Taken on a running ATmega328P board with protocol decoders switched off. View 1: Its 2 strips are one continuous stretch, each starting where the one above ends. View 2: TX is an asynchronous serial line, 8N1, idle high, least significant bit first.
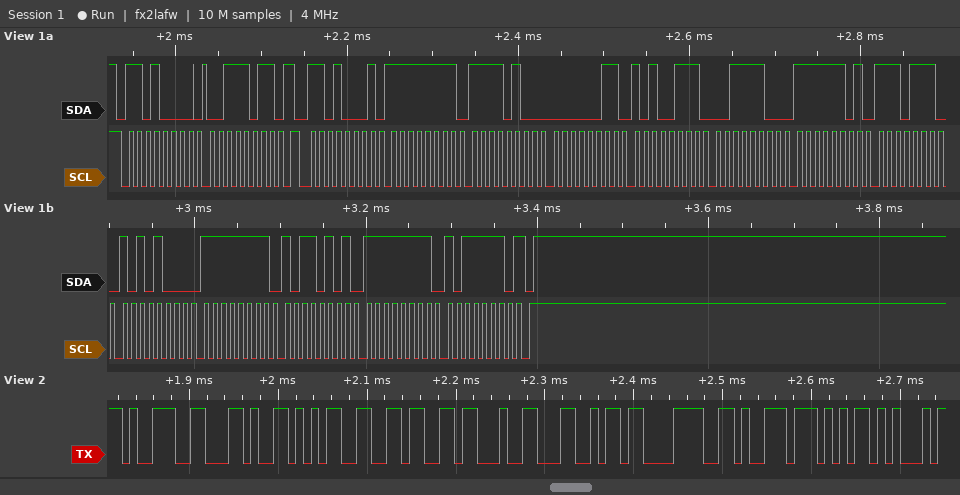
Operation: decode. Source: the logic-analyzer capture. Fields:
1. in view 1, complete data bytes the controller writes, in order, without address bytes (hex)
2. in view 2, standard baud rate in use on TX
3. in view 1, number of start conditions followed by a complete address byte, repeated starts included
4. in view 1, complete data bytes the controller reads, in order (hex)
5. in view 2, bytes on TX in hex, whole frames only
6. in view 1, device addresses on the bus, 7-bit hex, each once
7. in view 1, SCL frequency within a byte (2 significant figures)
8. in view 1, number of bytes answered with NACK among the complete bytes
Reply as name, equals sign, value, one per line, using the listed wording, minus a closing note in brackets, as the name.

in view 1, complete data bytes the controller writes, in order, without address bytes = 3B
in view 2, standard baud rate in use on TX = 115200 baud
in view 1, number of start conditions followed by a complete address byte, repeated starts included = 2
in view 1, complete data bytes the controller reads, in order = FF F4 03 A7 3C FD EE A8 FF B5 FF BE
in view 2, bytes on TX in hex, whole frames only = 39 2C 35 36 23 4C C3 96 57 45
in view 1, device addresses on the bus, 7-bit hex, each once = 0x68
in view 1, SCL frequency within a byte = 100 kHz
in view 1, number of bytes answered with NACK among the complete bytes = 1
